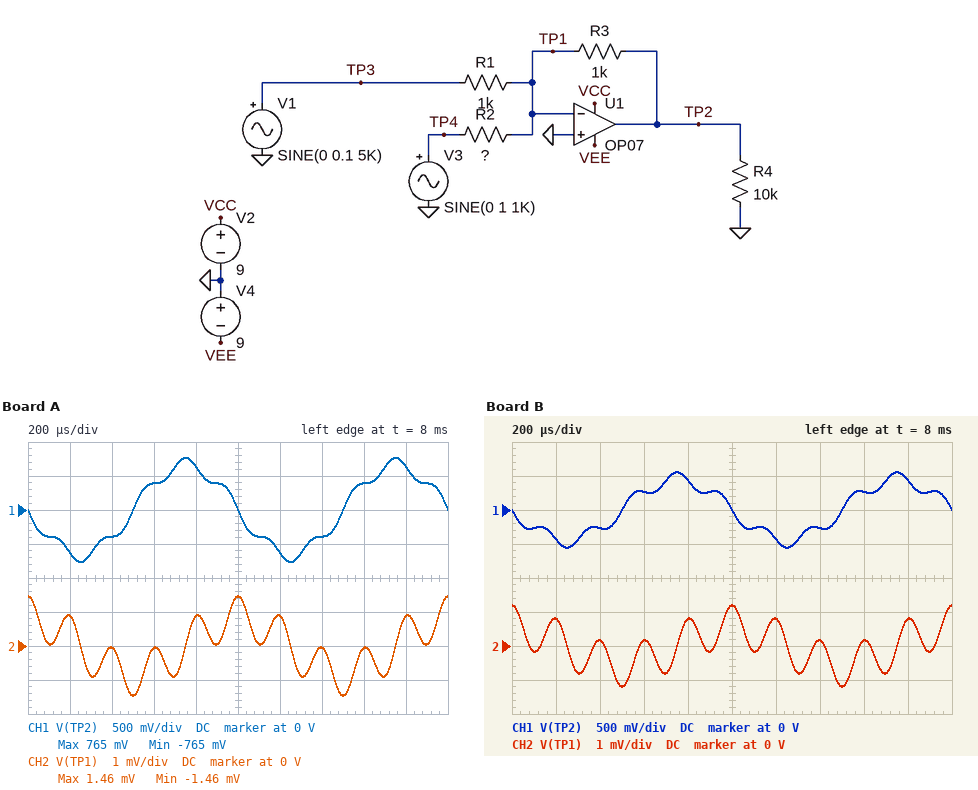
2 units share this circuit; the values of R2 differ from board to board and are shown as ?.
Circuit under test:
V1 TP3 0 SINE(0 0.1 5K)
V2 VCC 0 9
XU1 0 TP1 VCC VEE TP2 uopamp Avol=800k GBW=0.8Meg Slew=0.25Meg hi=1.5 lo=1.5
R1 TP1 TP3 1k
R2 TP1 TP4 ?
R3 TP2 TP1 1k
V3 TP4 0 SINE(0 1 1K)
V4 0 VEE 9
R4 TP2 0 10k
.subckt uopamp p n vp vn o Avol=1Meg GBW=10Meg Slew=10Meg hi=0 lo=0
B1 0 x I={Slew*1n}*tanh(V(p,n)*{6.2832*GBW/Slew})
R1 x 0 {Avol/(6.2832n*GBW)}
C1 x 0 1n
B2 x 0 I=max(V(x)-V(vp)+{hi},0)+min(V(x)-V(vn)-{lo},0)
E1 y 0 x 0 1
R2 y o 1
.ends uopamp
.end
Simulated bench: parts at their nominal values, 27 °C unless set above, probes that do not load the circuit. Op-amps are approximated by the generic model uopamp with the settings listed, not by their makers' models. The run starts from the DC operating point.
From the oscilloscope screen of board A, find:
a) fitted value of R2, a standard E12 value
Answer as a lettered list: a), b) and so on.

a) 1.5 kΩ
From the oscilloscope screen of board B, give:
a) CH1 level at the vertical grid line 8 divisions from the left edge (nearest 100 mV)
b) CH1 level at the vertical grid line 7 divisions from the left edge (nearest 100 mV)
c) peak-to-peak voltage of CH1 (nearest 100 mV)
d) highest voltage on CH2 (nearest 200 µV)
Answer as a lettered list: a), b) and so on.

a) 300 mV
b) -300 mV
c) 1.1 V
d) 1.2 mV
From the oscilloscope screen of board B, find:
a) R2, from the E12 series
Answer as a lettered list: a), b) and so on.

a) 2.2 kΩ
